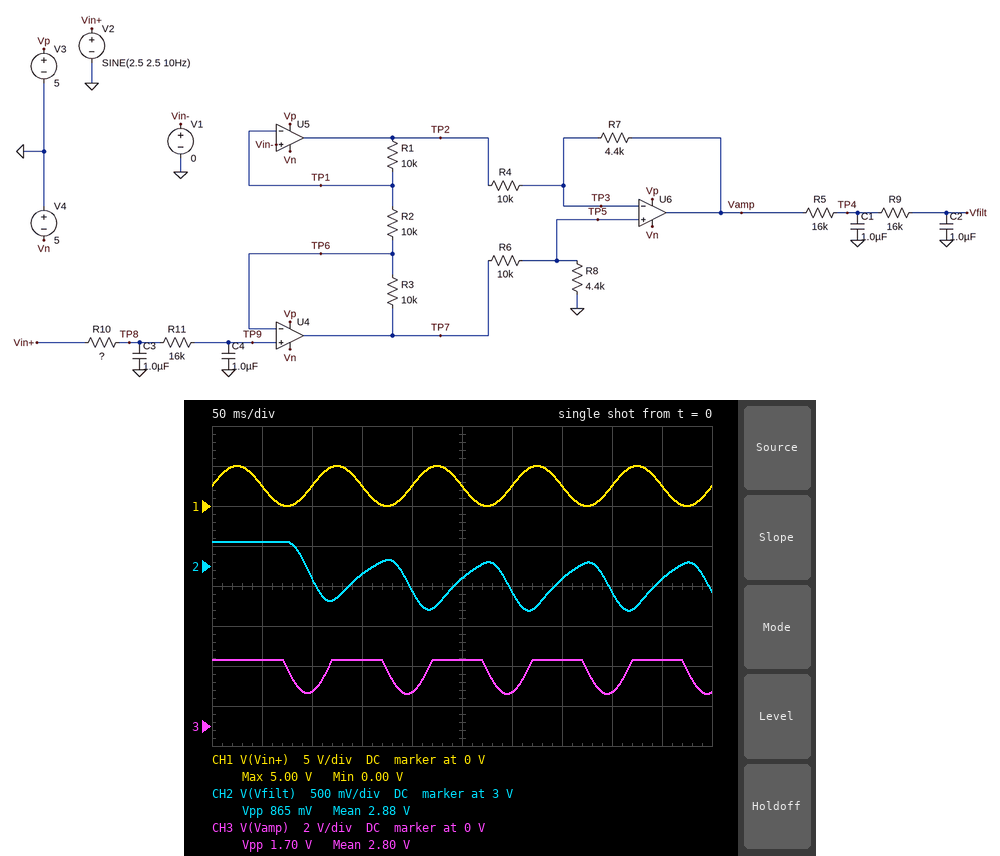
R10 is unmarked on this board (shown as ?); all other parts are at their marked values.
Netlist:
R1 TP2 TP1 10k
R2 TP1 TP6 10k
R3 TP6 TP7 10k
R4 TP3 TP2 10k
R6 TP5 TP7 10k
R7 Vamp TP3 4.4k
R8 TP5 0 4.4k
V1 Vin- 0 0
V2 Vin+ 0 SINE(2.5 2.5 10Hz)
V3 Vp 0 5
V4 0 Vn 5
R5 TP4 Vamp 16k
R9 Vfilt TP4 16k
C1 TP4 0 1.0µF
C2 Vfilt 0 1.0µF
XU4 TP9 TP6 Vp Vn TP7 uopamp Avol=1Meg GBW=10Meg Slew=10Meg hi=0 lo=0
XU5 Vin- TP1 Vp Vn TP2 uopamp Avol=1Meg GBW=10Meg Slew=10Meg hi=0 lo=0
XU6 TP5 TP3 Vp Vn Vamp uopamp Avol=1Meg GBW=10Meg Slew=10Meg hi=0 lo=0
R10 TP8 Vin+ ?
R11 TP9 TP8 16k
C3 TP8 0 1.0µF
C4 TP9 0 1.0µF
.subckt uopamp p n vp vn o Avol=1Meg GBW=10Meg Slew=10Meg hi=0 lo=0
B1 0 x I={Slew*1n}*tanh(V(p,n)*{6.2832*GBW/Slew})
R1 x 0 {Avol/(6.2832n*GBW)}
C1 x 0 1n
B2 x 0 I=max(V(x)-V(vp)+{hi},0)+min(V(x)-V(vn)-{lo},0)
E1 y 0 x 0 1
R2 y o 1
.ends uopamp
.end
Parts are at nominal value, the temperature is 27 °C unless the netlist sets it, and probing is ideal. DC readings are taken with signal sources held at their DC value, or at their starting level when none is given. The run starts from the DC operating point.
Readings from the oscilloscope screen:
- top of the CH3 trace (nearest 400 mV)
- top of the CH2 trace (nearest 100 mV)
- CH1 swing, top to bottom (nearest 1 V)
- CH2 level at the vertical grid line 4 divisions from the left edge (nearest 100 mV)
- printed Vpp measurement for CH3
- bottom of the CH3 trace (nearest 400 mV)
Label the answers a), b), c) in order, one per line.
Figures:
a) 3.2 V
b) 3.3 V
c) 5 V
d) 2.7 V
e) 1.70 V
f) 1.6 V
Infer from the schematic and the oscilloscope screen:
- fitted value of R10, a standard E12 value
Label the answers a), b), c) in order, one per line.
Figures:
a) 6.8 kΩ
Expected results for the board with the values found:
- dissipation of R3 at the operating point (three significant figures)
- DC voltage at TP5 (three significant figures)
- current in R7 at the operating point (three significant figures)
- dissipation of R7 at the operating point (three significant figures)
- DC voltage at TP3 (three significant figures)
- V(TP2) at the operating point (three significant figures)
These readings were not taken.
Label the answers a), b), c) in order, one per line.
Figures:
a) 625 µW
b) 1.53 V
c) 403 µA
d) 714 µW
e) 1.53 V
f) -2.50 V
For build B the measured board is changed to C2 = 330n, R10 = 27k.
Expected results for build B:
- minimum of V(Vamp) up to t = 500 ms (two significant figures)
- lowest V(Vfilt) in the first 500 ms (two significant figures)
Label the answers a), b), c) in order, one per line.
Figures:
a) 2.6 V
b) 2.8 V
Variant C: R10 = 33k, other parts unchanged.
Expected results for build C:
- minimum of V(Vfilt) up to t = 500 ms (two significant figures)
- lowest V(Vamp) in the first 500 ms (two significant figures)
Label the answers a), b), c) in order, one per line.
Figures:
a) 3.0 V
b) 2.7 V
